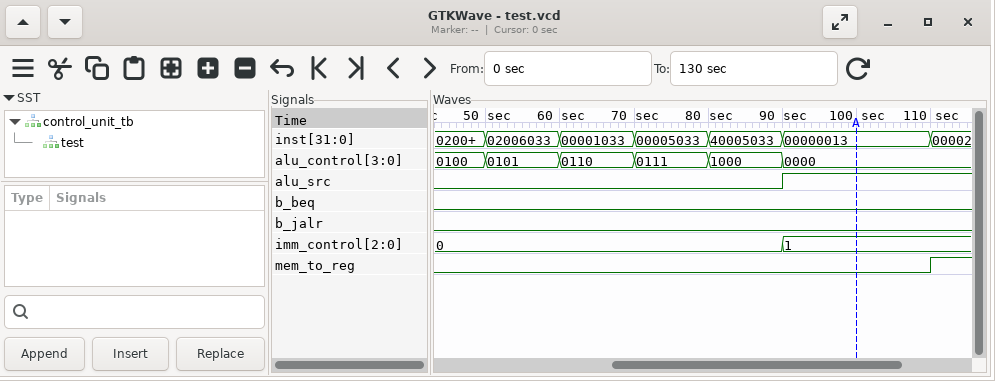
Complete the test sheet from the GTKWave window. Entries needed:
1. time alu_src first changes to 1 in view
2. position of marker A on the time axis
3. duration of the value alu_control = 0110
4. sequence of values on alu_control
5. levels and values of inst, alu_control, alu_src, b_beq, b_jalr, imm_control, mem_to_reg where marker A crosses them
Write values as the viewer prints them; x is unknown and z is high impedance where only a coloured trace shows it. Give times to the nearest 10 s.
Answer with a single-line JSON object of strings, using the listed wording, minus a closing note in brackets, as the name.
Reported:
{"time alu_src first changes to 1 in view": "90 s", "position of marker A on the time axis": "100 s", "duration of the value alu_control = 0110": "10 s", "sequence of values on alu_control": "0100, 0101, 0110, 0111, 1000, 0000", "levels and values of inst, alu_control, alu_src, b_beq, b_jalr, imm_control, mem_to_reg where marker A crosses them": "inst=00000013, alu_control=0000, alu_src=1, b_beq=0, b_jalr=0, imm_control=1, mem_to_reg=0"}
